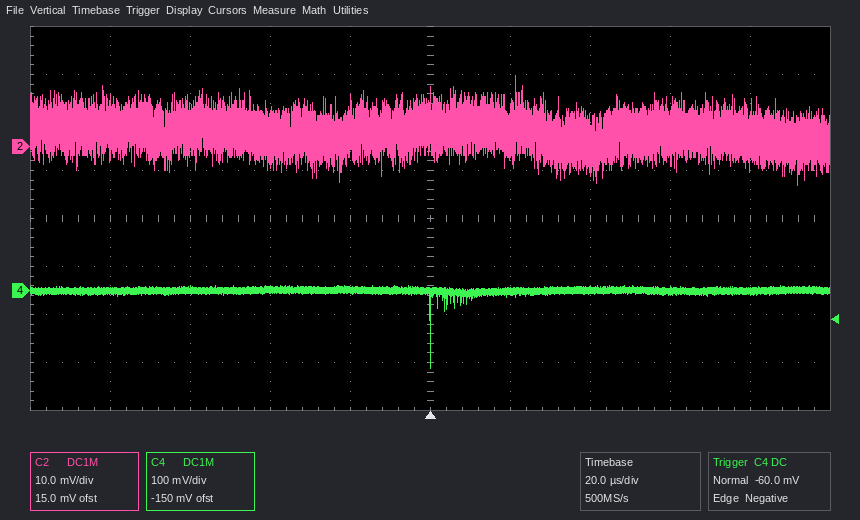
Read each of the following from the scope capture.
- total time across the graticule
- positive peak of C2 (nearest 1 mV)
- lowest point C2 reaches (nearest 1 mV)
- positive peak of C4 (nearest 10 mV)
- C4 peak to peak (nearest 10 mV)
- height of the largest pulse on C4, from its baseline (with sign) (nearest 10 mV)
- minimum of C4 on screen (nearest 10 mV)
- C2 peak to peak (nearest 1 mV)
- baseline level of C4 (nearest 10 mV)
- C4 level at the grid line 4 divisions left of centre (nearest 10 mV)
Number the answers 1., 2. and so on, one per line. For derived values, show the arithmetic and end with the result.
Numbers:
1. 200 µs
2. 15 mV
3. -8 mV
4. 10 mV
5. 10 mV − (-160 mV) = 170 mV
6. -160 mV − (0 mV) = -160 mV
7. -160 mV
8. 15 mV − (-8 mV) = 23 mV
9. 0 mV
10. 0 mV
